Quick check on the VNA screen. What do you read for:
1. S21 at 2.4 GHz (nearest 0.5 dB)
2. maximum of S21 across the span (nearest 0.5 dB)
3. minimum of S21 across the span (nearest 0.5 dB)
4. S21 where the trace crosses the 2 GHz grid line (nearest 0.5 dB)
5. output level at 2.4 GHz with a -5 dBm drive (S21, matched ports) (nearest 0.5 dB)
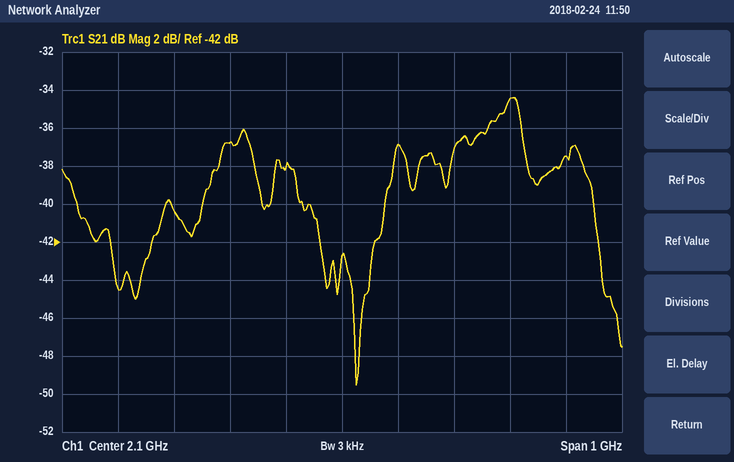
-34.5 dB
-34.5 dB
-49.5 dB
-38.0 dB
-39.5 dBm
